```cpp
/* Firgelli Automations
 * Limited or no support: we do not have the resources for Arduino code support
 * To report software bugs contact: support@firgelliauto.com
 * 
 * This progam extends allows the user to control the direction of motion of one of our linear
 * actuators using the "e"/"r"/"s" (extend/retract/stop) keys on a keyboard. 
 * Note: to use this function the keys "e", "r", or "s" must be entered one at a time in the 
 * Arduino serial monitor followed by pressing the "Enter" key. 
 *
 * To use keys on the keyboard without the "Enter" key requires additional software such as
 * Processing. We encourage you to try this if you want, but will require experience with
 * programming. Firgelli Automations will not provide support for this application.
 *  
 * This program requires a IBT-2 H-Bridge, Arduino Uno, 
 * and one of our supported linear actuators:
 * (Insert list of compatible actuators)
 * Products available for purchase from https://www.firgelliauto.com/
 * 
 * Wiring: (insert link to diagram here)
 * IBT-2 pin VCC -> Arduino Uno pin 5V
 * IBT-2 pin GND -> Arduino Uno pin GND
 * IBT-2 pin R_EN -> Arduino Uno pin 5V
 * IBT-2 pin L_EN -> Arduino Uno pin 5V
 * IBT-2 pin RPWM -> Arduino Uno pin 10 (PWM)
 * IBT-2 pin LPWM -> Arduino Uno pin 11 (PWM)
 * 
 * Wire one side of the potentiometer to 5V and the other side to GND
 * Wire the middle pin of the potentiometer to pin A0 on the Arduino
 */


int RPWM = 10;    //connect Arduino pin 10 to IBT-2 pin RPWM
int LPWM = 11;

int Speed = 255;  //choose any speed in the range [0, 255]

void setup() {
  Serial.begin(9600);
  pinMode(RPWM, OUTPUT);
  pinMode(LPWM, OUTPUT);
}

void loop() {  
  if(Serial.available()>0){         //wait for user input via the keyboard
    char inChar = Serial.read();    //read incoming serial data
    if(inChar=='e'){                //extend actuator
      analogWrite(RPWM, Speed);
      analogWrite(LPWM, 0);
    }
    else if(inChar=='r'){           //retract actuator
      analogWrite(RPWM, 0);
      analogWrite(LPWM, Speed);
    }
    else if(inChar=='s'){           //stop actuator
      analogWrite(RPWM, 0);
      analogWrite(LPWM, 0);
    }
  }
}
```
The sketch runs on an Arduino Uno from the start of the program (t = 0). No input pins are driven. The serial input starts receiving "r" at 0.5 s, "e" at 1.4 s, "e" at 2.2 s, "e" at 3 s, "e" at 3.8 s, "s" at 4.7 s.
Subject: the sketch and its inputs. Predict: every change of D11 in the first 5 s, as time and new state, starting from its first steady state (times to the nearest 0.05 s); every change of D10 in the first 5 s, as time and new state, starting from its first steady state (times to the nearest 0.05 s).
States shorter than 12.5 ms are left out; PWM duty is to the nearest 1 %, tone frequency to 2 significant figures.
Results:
0 s low; 0.5 s high; 1.4 s low
0 s low; 1.4 s high; 4.7 s low
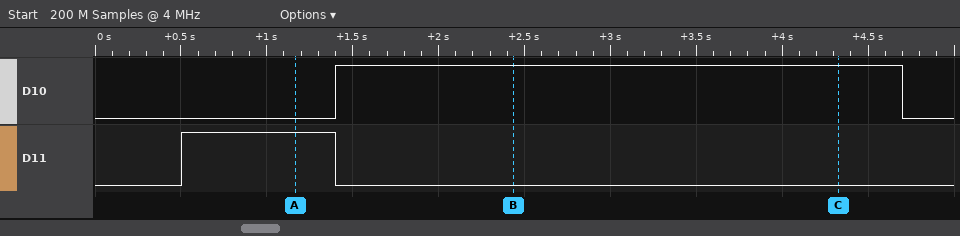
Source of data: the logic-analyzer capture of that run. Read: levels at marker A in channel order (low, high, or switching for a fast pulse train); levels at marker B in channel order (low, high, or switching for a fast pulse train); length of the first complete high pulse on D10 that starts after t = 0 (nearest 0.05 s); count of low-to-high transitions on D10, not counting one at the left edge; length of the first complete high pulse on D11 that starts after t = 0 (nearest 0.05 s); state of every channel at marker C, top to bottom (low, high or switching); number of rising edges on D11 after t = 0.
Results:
D10 low, D11 high
D10 high, D11 low
3.30 s
1
0.90 s
D10 high, D11 low
1
